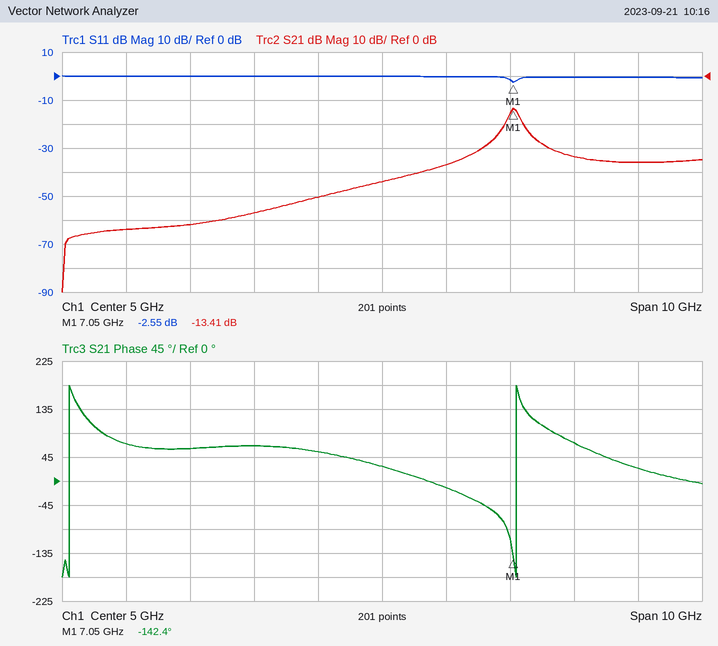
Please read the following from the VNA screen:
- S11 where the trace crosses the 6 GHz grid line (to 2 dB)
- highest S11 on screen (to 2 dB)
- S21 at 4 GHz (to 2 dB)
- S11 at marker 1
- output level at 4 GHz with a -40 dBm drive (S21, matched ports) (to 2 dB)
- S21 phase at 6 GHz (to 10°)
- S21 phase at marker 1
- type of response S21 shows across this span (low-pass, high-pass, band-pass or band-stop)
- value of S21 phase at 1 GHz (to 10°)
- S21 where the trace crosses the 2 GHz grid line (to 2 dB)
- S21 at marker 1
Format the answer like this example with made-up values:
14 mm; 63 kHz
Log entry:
0 dB; 0 dB; -50 dB; -2.55 dB; -90 dBm; -10°; -142.4°; band-pass; 70°; -62 dB; -13.41 dB
